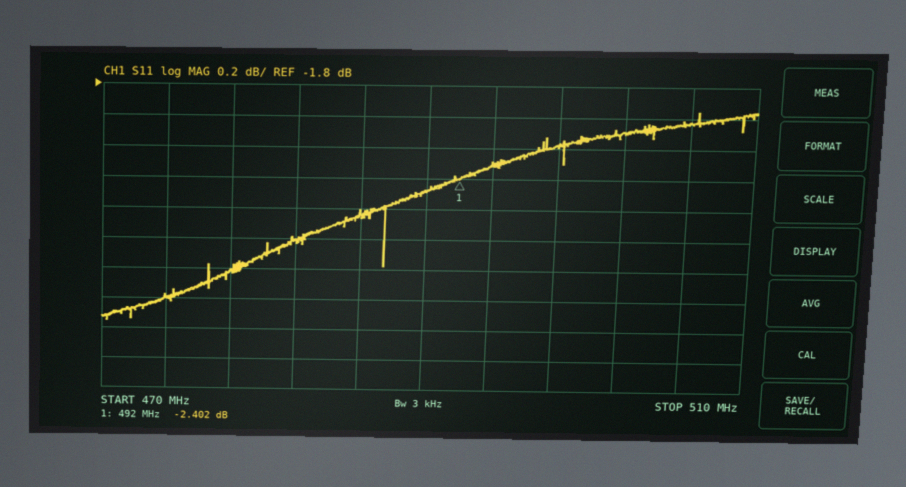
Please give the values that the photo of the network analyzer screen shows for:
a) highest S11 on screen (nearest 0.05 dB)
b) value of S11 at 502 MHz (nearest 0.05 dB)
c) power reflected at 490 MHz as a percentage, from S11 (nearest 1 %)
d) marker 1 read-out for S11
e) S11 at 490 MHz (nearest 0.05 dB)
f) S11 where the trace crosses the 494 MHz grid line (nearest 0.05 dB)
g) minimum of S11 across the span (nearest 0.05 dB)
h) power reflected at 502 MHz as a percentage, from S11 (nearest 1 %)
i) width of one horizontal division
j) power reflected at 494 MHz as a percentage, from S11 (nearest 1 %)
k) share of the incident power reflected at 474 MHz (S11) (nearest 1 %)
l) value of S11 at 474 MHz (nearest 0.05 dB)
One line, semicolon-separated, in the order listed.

-1.95 dB; -2.10 dB; 56 %; -2.402 dB; -2.50 dB; -2.30 dB; -3.35 dB; 62 %; 4 MHz; 59 %; 48 %; -3.20 dB
